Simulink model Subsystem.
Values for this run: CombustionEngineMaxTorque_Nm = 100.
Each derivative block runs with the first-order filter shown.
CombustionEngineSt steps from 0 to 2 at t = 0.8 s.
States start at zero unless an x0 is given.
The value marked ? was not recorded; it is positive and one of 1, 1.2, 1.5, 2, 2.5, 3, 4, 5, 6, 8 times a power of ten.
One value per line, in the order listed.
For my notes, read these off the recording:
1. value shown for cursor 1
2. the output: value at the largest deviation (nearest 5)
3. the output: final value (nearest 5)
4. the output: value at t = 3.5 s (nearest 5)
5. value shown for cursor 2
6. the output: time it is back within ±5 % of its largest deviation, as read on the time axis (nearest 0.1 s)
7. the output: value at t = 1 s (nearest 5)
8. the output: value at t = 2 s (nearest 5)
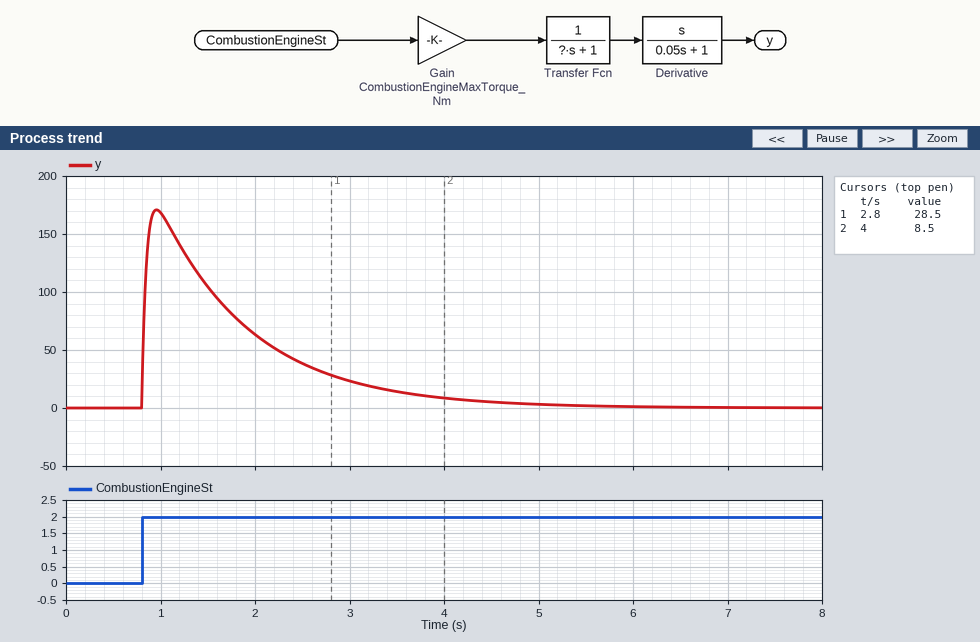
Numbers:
28.5
170
0
15
8.5
4.0 s
170
65
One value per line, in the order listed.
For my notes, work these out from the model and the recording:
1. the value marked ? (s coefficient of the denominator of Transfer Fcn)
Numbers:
1
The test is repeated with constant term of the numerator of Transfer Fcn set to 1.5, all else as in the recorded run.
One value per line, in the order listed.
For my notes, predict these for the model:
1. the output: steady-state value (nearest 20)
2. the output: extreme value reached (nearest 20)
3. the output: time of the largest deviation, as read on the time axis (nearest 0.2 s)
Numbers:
0
260
1.0 s
